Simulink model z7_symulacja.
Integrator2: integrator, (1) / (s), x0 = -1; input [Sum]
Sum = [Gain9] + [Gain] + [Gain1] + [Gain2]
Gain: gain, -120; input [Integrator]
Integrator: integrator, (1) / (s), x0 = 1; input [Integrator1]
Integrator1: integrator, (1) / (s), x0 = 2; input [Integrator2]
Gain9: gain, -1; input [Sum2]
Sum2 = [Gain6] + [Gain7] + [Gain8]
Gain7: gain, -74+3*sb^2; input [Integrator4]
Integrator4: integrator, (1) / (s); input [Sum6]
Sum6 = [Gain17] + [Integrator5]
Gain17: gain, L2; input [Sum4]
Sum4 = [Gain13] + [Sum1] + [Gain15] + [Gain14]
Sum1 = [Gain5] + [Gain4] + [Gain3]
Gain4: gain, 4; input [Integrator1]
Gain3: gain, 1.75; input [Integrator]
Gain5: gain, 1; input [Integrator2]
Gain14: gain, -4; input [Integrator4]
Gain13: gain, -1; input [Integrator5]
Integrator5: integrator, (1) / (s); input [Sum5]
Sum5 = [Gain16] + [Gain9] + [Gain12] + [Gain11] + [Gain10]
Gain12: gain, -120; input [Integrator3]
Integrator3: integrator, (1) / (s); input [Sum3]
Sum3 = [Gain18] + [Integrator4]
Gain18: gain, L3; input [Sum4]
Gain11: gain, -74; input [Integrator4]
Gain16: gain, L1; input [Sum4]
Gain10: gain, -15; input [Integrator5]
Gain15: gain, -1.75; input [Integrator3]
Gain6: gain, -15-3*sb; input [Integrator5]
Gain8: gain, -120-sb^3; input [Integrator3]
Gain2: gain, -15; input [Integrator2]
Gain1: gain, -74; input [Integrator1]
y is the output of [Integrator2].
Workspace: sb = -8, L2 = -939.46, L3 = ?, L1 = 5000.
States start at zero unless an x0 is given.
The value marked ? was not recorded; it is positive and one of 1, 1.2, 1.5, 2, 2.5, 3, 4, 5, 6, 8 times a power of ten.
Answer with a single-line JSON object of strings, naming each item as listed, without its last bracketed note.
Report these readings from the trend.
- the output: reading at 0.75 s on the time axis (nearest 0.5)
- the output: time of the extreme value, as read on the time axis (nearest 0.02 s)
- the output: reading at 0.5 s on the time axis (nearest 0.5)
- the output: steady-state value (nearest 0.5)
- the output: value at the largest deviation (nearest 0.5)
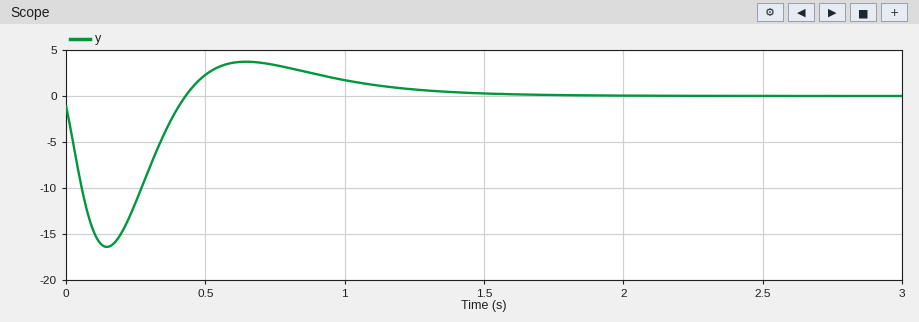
{"the output: reading at 0.75 s on the time axis": "3.5", "the output: time of the extreme value, as read on the time axis": "0.14 s", "the output: reading at 0.5 s on the time axis": "2.5", "the output: steady-state value": "0.0", "the output: value at the largest deviation": "-16.5"}
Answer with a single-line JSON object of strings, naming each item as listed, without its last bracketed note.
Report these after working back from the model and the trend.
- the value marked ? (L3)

{"the value marked ?": "120"}
